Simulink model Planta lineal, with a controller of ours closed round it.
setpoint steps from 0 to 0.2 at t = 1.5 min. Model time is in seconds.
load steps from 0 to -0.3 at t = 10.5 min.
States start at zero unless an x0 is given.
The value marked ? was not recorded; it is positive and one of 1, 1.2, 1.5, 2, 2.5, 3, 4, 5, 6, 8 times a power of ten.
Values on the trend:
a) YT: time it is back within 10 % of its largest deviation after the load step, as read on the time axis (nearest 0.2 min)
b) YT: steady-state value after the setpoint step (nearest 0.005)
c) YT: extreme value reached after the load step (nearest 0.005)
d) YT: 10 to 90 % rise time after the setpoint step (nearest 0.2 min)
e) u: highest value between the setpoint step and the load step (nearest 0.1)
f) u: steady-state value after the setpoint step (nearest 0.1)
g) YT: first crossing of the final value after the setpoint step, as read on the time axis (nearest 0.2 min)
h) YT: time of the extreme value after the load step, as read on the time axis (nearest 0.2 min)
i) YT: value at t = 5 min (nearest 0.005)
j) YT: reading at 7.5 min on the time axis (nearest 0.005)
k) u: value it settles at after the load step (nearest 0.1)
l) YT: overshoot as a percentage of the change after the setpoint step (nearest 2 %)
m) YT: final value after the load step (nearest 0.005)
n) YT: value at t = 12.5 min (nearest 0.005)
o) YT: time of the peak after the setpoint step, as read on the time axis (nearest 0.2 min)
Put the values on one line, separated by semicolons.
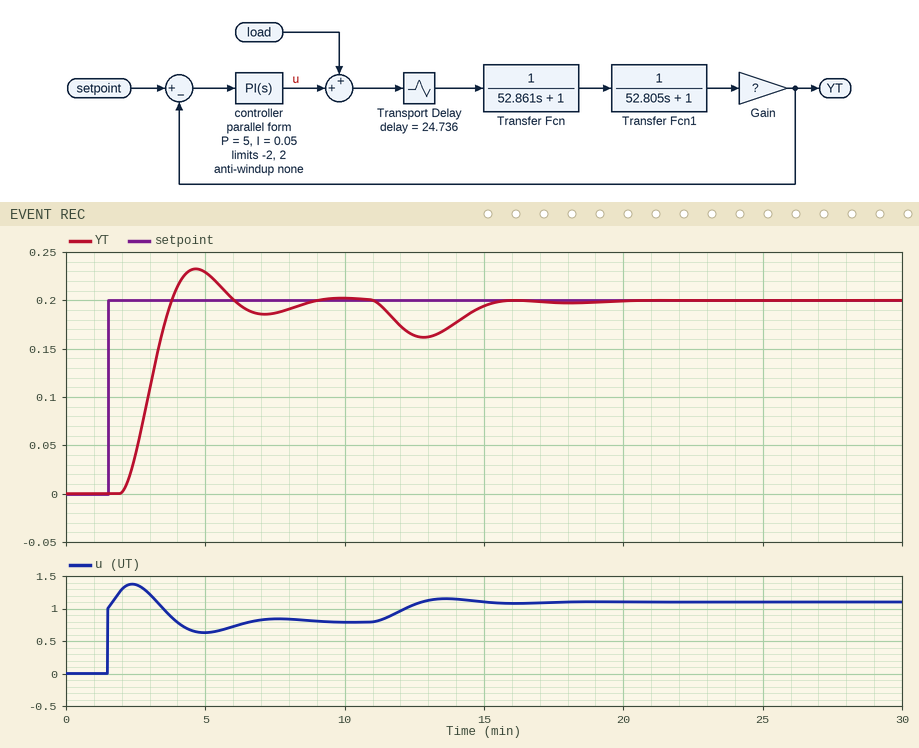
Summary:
15.2 min; 0.200; 0.160; 1.2 min; 1.4; 0.8; 3.8 min; 12.8 min; 0.230; 0.185; 1.1; 16 %; 0.200; 0.165; 4.6 min
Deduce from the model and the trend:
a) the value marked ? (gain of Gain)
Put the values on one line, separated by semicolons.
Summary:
0.25
